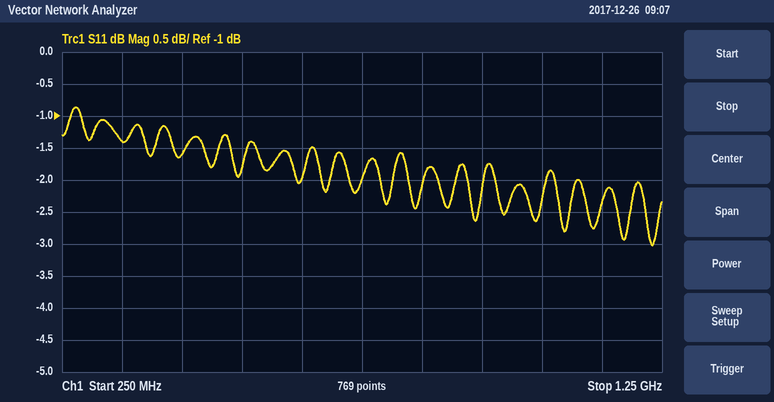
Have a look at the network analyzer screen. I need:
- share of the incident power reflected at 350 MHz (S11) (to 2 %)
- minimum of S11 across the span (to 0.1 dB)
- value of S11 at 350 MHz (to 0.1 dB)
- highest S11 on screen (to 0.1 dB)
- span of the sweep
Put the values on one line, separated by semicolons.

72 %; -3.0 dB; -1.4 dB; -0.9 dB; 1 GHz
